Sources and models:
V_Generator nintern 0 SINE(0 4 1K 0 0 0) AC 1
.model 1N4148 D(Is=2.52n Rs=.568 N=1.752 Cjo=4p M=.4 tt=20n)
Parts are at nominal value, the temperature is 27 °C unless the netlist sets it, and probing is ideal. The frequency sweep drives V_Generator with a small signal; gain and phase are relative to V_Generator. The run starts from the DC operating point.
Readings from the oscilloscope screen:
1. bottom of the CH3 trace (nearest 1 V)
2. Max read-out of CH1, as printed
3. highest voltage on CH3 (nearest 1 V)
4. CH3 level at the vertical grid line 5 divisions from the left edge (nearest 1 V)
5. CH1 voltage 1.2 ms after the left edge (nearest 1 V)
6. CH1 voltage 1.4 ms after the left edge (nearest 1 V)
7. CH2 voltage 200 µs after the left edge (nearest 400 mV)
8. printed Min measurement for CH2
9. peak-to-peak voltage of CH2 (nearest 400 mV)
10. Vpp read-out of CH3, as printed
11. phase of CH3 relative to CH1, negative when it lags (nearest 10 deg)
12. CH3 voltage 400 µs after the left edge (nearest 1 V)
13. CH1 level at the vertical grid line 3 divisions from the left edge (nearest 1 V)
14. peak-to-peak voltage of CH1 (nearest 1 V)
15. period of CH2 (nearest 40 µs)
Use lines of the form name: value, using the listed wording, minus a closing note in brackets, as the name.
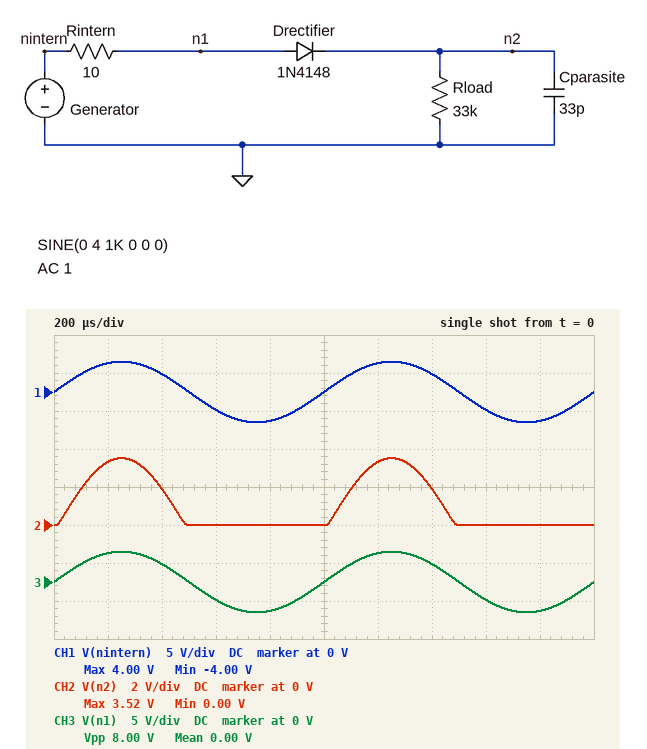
bottom of the CH3 trace: -4 V
Max read-out of CH1, as printed: 4.00 V
highest voltage on CH3: 4 V
CH3 level at the vertical grid line 5 divisions from the left edge: 0 V
CH1 voltage 1.2 ms after the left edge: 4 V
CH1 voltage 1.4 ms after the left edge: 2 V
CH2 voltage 200 µs after the left edge: 3.2 V
printed Min measurement for CH2: 0.00 V
peak-to-peak voltage of CH2: 3.6 V
Vpp read-out of CH3, as printed: 8.00 V
phase of CH3 relative to CH1, negative when it lags: 0 deg
CH3 voltage 400 µs after the left edge: 2 V
CH1 level at the vertical grid line 3 divisions from the left edge: -2 V
peak-to-peak voltage of CH1: 8 V
period of CH2: 1.00 ms
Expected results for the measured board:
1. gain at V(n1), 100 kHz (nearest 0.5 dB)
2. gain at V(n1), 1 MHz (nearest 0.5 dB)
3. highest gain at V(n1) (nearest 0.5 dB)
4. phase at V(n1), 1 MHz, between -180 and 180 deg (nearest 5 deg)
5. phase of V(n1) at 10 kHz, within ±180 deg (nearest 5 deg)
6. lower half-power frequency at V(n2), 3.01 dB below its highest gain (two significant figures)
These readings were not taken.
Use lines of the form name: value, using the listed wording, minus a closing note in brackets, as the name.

gain at V(n1), 100 kHz: 0 dB
gain at V(n1), 1 MHz: 0 dB
highest gain at V(n1): 0 dB
phase at V(n1), 1 MHz, between -180 and 180 deg: 0 deg
phase of V(n1) at 10 kHz, within ±180 deg: 0 deg
lower half-power frequency at V(n2), 3.01 dB below its highest gain: 130 kHz
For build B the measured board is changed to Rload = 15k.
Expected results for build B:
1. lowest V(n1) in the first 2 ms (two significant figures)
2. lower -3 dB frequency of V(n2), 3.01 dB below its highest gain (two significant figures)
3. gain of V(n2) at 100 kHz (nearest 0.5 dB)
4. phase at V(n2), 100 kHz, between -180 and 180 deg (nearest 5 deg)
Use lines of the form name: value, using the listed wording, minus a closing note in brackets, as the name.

lowest V(n1) in the first 2 ms: -4.0 V
lower -3 dB frequency of V(n2), 3.01 dB below its highest gain: 290 kHz
gain of V(n2) at 100 kHz: -29.0 dB
phase at V(n2), 100 kHz, between -180 and 180 deg: 70 deg
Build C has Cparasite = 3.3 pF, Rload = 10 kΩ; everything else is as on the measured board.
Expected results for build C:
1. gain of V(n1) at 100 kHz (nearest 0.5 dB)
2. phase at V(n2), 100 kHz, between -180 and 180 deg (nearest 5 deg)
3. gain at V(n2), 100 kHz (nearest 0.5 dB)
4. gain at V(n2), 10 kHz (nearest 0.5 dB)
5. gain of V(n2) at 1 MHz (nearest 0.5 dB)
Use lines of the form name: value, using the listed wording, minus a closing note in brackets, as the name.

gain of V(n1) at 100 kHz: 0 dB
phase at V(n2), 100 kHz, between -180 and 180 deg: 85 deg
gain at V(n2), 100 kHz: -32.0 dB
gain at V(n2), 10 kHz: -52.0 dB
gain of V(n2) at 1 MHz: -13.0 dB
